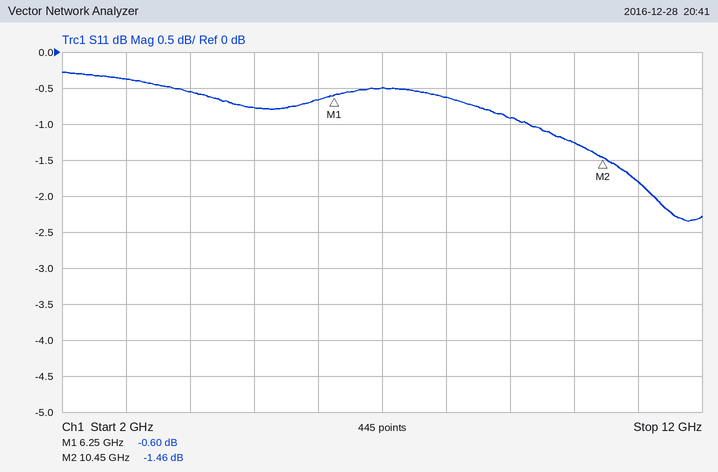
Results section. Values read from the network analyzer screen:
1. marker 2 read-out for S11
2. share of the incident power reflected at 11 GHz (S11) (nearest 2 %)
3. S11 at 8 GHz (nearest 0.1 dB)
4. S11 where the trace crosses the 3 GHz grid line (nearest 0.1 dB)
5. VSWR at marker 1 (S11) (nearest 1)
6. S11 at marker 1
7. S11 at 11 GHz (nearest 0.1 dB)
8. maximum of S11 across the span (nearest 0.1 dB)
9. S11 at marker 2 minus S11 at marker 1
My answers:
-1.46 dB
66 %
-0.6 dB
-0.4 dB
29
-0.60 dB
-1.8 dB
-0.3 dB
-0.86 dB
